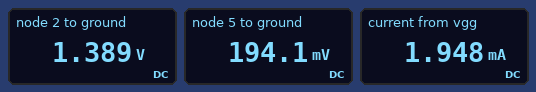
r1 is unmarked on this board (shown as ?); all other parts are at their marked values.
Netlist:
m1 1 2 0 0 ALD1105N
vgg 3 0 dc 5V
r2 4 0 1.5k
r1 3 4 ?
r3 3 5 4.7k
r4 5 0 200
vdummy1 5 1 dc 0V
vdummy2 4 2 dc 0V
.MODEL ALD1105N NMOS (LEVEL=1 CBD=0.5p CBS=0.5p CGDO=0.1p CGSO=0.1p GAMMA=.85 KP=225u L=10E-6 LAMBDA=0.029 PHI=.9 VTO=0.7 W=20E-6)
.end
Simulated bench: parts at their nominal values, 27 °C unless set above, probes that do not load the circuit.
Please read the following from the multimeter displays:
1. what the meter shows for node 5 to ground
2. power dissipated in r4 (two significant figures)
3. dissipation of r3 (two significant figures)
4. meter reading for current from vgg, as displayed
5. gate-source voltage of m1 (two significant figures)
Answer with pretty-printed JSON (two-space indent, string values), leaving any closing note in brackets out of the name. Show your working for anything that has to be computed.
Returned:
{
  "what the meter shows for node 5 to ground": "194.1 mV",
  "power dissipated in r4": "(194.1 mV)^2 / 200 Ω = 190 µW",
  "dissipation of r3": "(5 V - 194.1 mV)^2 / 4.7 kΩ = 4.9 mW",
  "meter reading for current from vgg, as displayed": "1.948 mA",
  "gate-source voltage of m1": "1.389 V = 1.4 V"
}
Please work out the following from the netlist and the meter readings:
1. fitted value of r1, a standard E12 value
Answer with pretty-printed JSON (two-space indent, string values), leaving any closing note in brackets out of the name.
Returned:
{
  "fitted value of r1, a standard E12 value": "3.9 kΩ"
}
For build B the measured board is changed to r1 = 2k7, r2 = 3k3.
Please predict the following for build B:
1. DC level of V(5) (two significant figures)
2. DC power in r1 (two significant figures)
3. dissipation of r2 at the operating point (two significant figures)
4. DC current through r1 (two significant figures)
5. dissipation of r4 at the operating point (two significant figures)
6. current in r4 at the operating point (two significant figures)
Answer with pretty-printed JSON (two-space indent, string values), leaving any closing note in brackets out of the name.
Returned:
{
  "DC level of V(5)": "170 mV",
  "DC power in r1": "1.9 mW",
  "dissipation of r2 at the operating point": "2.3 mW",
  "DC current through r1": "830 µA",
  "dissipation of r4 at the operating point": "150 µW",
  "current in r4 at the operating point": "870 µA"
}
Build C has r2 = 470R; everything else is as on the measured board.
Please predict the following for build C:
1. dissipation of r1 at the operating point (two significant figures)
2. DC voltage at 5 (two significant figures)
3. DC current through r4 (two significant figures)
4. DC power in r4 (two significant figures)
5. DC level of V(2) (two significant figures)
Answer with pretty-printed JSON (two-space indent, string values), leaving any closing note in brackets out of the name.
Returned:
{
  "dissipation of r1 at the operating point": "5.1 mW",
  "DC voltage at 5": "200 mV",
  "DC current through r4": "1.0 mA",
  "DC power in r4": "210 µW",
  "DC level of V(2)": "540 mV"
}
